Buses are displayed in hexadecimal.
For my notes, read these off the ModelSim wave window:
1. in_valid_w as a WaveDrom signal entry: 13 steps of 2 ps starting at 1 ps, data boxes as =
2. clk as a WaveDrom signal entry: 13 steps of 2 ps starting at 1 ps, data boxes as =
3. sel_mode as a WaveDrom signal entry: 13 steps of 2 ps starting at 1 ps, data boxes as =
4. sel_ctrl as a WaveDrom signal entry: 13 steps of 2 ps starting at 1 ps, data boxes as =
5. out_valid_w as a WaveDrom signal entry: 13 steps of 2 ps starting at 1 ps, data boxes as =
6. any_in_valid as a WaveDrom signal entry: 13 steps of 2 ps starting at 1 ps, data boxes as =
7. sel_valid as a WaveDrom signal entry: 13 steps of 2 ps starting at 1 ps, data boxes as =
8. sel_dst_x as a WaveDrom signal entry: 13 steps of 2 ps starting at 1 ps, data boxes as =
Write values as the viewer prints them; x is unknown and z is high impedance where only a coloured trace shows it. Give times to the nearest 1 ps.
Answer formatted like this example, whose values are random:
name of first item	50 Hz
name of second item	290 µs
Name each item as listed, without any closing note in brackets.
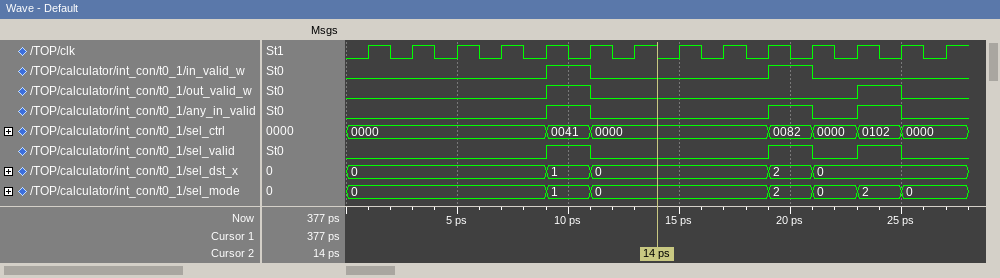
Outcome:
in_valid_w as a WaveDrom signal entry: 13 steps of 2 ps starting at 1 ps, data boxes as =	{name: 'in_valid_w', wave: '0...10...10..'}
clk as a WaveDrom signal entry: 13 steps of 2 ps starting at 1 ps, data boxes as =	{name: 'clk', wave: 'p............'}
sel_mode as a WaveDrom signal entry: 13 steps of 2 ps starting at 1 ps, data boxes as =	{name: 'sel_mode', wave: '=...==...====', data: '0 1 0 2 0 2 0'}
sel_ctrl as a WaveDrom signal entry: 13 steps of 2 ps starting at 1 ps, data boxes as =	{name: 'sel_ctrl', wave: '=...==...====', data: '0000 0041 0000 0082 0000 0102 0000'}
out_valid_w as a WaveDrom signal entry: 13 steps of 2 ps starting at 1 ps, data boxes as =	{name: 'out_valid_w', wave: '0...10.....10'}
any_in_valid as a WaveDrom signal entry: 13 steps of 2 ps starting at 1 ps, data boxes as =	{name: 'any_in_valid', wave: '0...10...1010'}
sel_valid as a WaveDrom signal entry: 13 steps of 2 ps starting at 1 ps, data boxes as =	{name: 'sel_valid', wave: '0...10...1010'}
sel_dst_x as a WaveDrom signal entry: 13 steps of 2 ps starting at 1 ps, data boxes as =	{name: 'sel_dst_x', wave: '=...==...==..', data: '0 1 0 2 0'}
